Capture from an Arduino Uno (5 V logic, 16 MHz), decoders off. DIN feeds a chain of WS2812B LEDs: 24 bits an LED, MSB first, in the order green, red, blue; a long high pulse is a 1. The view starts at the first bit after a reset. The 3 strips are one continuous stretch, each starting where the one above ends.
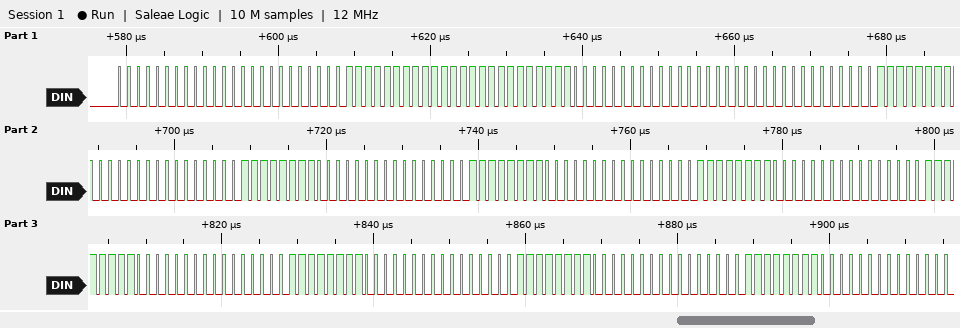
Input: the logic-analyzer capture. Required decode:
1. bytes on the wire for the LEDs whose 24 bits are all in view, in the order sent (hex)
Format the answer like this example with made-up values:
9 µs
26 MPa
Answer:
00 00 00 FF FF FF 00 00 00 00 FF 00 00 FF 00 00 FF 00 00 FF 00 00 FF 00 00 FF 00 00 FF 00 00 FF 00
